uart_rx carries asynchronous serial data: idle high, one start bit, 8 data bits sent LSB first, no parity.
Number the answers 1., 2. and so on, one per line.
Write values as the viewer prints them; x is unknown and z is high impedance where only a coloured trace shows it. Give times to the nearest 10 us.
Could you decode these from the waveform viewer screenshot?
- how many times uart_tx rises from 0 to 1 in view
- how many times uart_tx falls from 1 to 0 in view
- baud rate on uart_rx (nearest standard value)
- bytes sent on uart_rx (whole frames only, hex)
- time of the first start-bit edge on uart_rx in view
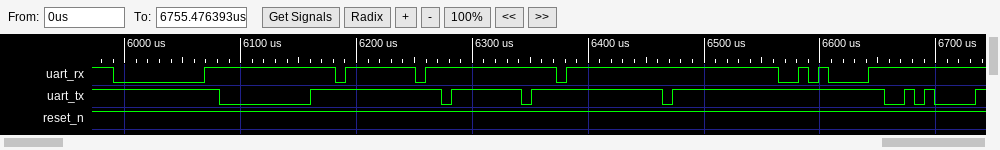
1. 7
2. 7
3. 115200 baud
4. 00, 7F, FF, 0A
5. 5990 us
